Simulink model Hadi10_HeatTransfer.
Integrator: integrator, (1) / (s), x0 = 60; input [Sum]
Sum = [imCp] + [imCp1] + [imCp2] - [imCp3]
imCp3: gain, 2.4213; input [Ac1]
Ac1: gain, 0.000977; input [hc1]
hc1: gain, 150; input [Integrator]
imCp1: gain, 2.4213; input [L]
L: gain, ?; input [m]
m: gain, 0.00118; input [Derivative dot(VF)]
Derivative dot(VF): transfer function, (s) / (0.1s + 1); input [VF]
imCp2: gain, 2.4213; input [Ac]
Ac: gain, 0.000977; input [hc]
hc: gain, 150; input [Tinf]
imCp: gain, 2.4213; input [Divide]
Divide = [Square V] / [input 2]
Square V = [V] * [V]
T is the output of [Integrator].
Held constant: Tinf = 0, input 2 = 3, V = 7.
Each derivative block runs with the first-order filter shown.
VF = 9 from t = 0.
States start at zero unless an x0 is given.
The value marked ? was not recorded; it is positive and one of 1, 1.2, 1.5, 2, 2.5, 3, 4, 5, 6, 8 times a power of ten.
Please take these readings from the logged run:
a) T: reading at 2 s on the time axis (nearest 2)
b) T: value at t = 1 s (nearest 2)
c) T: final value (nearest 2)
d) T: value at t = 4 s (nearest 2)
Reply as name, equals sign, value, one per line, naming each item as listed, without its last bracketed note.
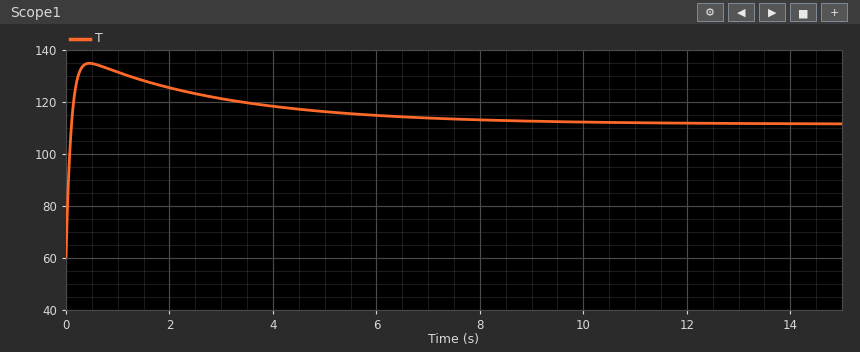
T: reading at 2 s on the time axis = 126
T: value at t = 1 s = 132
T: final value = 112
T: value at t = 4 s = 118
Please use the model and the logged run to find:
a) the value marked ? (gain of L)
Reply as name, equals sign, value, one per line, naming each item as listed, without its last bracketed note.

the value marked ? = 3000
